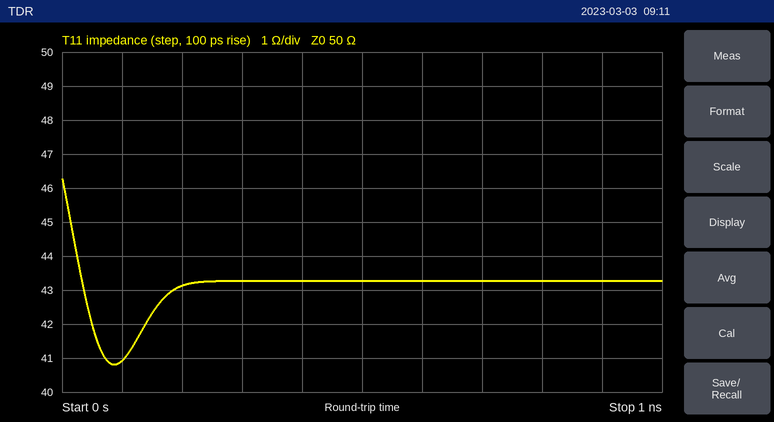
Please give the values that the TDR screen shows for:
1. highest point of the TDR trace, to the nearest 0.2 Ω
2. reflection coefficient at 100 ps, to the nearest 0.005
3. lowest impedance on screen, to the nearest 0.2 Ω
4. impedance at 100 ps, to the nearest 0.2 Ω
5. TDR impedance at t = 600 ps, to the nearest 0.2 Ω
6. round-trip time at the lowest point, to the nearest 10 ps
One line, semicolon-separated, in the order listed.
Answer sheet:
46.2 Ω; -0.100; 40.8 Ω; 41.0 Ω; 43.2 Ω; 90 ps
